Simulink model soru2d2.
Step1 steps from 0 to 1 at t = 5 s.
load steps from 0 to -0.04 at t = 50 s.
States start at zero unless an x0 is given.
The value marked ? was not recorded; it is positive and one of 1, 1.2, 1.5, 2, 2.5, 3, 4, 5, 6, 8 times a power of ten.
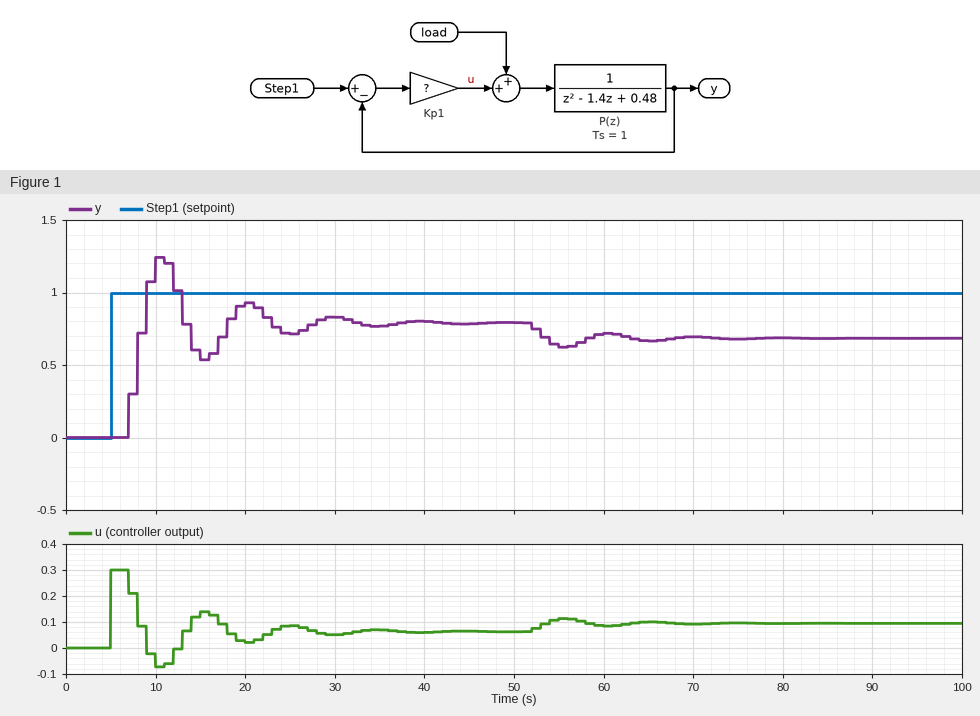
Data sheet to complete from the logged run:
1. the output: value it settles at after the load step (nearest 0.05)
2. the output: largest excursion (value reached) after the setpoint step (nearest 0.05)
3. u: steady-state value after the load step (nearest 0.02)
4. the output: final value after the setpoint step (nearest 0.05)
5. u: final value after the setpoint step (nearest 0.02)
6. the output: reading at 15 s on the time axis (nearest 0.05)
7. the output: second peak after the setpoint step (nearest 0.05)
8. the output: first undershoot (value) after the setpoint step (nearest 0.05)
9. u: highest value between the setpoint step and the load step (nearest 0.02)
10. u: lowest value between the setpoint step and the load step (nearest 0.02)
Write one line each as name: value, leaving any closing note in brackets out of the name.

the output: value it settles at after the load step: 0.70
the output: largest excursion (value reached) after the setpoint step: 1.25
u: steady-state value after the load step: 0.10
the output: final value after the setpoint step: 0.80
u: final value after the setpoint step: 0.06
the output: reading at 15 s on the time axis: 0.55
the output: second peak after the setpoint step: 0.95
the output: first undershoot (value) after the setpoint step: 0.55
u: highest value between the setpoint step and the load step: 0.30
u: lowest value between the setpoint step and the load step: -0.08
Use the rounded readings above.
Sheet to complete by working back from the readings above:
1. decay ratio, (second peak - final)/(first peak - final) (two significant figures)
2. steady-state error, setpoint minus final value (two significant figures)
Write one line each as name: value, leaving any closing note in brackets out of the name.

decay ratio, (second peak - final)/(first peak - final): 0.33
steady-state error, setpoint minus final value: 0.20
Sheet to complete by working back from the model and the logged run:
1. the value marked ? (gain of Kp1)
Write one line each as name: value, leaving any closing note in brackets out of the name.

the value marked ?: 0.3
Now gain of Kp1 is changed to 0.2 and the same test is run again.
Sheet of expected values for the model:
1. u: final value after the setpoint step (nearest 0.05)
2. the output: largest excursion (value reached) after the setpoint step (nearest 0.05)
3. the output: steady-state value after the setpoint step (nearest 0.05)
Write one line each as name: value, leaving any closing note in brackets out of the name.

u: final value after the setpoint step: 0.05
the output: largest excursion (value reached) after the setpoint step: 0.95
the output: steady-state value after the setpoint step: 0.70
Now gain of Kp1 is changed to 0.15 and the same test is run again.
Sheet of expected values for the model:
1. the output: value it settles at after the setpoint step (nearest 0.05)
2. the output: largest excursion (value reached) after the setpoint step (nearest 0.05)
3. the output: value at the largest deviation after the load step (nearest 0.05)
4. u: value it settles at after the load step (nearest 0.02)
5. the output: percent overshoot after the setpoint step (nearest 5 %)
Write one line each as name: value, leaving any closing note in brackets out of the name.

the output: value it settles at after the setpoint step: 0.65
the output: largest excursion (value reached) after the setpoint step: 0.80
the output: value at the largest deviation after the load step: 0.45
u: value it settles at after the load step: 0.08
the output: percent overshoot after the setpoint step: 25 %
